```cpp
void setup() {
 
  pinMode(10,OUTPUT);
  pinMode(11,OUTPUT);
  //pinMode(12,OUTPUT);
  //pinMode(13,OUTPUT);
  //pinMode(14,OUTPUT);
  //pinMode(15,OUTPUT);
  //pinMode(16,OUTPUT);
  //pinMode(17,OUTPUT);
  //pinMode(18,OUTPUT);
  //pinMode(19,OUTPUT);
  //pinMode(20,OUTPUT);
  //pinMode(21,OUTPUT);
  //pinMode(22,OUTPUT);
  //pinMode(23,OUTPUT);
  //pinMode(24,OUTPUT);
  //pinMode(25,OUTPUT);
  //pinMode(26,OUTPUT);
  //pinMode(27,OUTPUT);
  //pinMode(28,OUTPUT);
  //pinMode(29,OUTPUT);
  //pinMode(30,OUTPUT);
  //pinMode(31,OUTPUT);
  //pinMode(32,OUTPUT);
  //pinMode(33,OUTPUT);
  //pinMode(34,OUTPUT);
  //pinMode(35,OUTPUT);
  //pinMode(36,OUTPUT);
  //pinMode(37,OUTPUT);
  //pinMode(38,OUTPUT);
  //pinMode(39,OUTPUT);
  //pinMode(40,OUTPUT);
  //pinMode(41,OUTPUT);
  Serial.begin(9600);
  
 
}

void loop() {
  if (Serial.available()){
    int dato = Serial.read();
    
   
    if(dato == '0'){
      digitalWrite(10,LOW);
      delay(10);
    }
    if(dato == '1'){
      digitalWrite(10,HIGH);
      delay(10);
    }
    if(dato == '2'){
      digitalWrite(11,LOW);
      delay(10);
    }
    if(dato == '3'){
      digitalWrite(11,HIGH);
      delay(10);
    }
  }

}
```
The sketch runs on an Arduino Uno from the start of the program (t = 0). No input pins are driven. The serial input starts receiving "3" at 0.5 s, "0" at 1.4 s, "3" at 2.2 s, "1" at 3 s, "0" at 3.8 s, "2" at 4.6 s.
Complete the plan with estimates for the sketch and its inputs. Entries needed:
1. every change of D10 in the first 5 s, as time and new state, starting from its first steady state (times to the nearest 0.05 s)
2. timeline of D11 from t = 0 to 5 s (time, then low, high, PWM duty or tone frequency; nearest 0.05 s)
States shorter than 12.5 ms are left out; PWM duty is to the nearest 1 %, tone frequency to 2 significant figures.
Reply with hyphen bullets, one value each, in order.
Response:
- 0 s low; 3 s high; 3.8 s low
- 0 s low; 0.5 s high; 4.6 s low
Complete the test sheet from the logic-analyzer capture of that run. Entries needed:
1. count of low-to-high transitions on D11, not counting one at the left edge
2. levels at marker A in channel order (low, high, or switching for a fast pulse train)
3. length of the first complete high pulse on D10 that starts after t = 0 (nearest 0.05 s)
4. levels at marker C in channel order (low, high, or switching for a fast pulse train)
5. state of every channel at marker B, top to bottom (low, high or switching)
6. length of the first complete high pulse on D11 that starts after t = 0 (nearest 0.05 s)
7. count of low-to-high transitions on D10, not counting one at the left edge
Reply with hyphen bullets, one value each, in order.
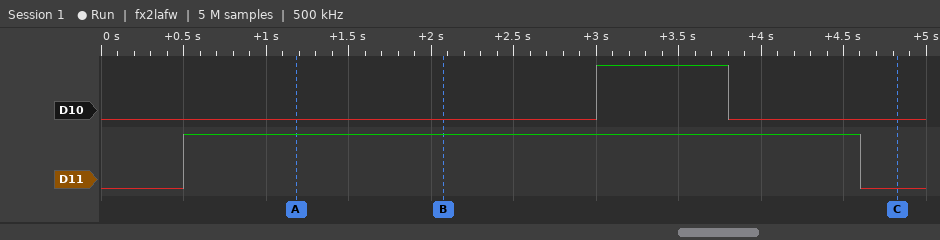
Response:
- 1
- D10 low, D11 high
- 0.80 s
- D10 low, D11 low
- D10 low, D11 high
- 4.10 s
- 1
